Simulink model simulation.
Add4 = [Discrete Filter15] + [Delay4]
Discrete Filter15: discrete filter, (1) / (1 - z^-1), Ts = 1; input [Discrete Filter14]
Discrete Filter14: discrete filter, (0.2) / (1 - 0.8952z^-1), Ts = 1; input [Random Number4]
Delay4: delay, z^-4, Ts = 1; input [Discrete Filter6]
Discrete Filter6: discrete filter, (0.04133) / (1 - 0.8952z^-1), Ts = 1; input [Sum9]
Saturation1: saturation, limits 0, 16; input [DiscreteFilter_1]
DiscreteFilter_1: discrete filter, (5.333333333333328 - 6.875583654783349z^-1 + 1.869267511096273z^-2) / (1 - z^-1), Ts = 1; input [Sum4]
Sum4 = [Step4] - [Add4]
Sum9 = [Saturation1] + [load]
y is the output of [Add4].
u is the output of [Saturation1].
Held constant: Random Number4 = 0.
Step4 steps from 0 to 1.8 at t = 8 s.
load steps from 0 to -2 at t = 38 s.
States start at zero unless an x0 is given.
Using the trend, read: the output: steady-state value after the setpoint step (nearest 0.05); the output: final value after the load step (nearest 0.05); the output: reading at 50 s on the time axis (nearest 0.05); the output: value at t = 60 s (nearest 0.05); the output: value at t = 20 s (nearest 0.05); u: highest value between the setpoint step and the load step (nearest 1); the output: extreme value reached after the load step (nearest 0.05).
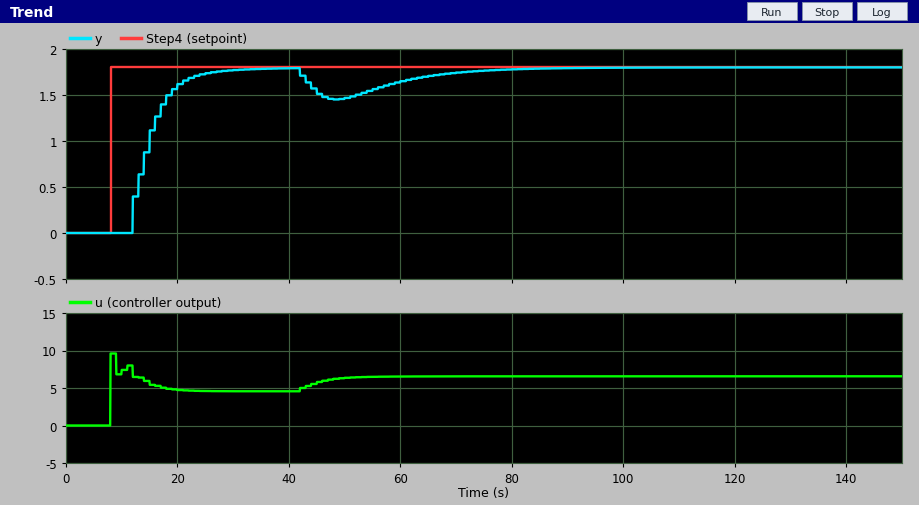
1.80
1.80
1.45
1.65
1.60
10
1.45
